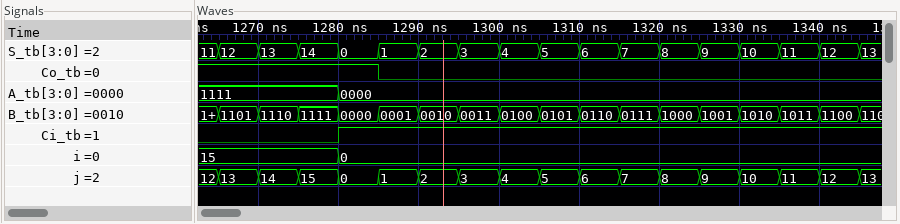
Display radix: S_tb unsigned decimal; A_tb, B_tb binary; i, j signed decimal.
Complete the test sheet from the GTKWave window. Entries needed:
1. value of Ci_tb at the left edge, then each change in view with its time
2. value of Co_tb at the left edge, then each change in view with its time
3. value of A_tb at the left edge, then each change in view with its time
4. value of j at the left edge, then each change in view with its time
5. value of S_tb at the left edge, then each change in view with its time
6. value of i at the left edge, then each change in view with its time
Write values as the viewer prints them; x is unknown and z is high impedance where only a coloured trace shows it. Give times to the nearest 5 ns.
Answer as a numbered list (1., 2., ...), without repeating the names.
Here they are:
1. 0, 1 at 1280 ns
2. 1, 0 at 1285 ns
3. 1111, 0000 at 1280 ns
4. 12, 13 at 1265 ns, 14 at 1270 ns, 15 at 1275 ns, 0 at 1280 ns, 1 at 1285 ns, 2 at 1290 ns, 3 at 1295 ns, 4 at 1300 ns, 5 at 1305 ns, 6 at 1310 ns, 7 at 1315 ns, 8 at 1320 ns, 9 at 1325 ns, 10 at 1330 ns, 11 at 1335 ns, 12 at 1340 ns, 13 at 1345 ns
5. 11, 12 at 1265 ns, 13 at 1270 ns, 14 at 1275 ns, 0 at 1280 ns, 1 at 1285 ns, 2 at 1290 ns, 3 at 1295 ns, 4 at 1300 ns, 5 at 1305 ns, 6 at 1310 ns, 7 at 1315 ns, 8 at 1320 ns, 9 at 1325 ns, 10 at 1330 ns, 11 at 1335 ns, 12 at 1340 ns, 13 at 1345 ns
6. 15, 0 at 1280 ns
